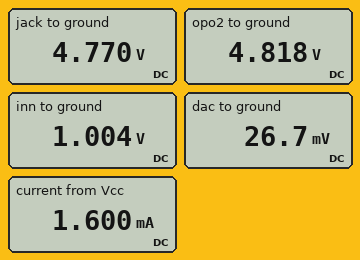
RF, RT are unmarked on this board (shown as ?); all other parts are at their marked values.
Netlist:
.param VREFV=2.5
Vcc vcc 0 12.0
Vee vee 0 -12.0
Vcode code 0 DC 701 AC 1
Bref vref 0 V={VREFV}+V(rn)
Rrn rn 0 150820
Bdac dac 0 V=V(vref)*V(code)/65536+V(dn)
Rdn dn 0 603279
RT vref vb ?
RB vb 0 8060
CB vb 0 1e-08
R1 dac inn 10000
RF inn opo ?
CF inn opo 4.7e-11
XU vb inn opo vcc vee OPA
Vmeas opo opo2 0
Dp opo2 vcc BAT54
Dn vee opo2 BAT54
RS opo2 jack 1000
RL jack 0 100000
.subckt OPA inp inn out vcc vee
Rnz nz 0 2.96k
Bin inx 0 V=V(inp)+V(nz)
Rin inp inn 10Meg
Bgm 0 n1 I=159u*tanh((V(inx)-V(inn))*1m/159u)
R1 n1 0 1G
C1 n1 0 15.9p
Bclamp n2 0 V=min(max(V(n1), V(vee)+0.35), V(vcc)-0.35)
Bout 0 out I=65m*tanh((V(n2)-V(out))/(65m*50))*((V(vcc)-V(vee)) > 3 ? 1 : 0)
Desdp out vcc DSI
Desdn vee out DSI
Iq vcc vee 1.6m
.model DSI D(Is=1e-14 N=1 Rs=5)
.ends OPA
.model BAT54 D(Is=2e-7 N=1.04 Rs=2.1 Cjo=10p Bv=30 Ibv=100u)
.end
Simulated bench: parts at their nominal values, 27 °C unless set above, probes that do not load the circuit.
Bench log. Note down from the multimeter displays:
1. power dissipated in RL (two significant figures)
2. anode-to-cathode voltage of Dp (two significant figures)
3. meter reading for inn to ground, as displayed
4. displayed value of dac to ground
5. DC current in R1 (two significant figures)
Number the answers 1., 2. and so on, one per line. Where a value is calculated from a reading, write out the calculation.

1. (4.77 V)^2 / 100 kΩ = 230 µW
2. 4.818 V - 12 V = -7.2 V
3. 1.004 V
4. 26.7 mV
5. (1.004 V - 26.7 mV) / 10 kΩ = 98 µA
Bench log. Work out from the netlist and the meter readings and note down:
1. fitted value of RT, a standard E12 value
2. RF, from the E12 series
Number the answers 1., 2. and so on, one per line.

1. 12 kΩ
2. 39 kΩ
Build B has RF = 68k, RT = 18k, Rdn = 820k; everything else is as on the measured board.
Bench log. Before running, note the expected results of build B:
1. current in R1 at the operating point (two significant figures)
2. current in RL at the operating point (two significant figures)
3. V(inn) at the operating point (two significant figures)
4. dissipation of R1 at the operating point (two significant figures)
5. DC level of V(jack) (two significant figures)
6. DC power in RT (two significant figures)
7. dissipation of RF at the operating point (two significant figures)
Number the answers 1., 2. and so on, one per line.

1. 75 µA
2. 58 µA
3. 770 mV
4. 56 µW
5. 5.8 V
6. 170 µW
7. 380 µW
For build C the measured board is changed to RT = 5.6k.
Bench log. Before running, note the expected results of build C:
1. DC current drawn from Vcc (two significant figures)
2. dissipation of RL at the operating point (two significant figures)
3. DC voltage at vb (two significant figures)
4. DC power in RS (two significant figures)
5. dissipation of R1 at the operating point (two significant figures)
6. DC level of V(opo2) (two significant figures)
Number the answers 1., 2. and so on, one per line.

1. 1.6 mA
2. 500 µW
3. 1.5 V
4. 5.0 µW
5. 210 µW
6. 7.1 V
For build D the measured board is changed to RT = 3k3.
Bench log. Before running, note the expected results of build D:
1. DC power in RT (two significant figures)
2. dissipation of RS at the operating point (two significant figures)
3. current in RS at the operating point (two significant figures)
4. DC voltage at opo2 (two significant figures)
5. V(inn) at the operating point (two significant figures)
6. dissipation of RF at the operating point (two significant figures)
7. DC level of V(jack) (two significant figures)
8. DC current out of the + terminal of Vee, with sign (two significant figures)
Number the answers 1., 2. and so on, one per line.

1. 160 µW
2. 7.2 µW
3. 85 µA
4. 8.6 V
5. 1.8 V
6. 1.2 mW
7. 8.5 V
8. -1.6 mA
